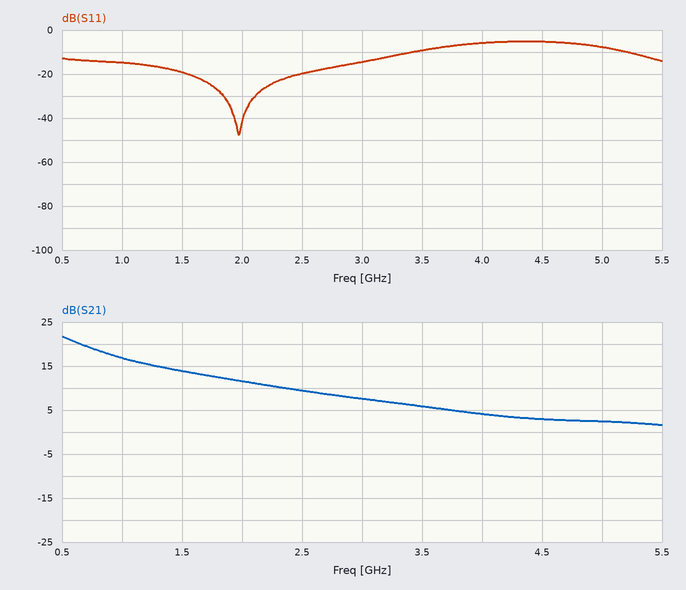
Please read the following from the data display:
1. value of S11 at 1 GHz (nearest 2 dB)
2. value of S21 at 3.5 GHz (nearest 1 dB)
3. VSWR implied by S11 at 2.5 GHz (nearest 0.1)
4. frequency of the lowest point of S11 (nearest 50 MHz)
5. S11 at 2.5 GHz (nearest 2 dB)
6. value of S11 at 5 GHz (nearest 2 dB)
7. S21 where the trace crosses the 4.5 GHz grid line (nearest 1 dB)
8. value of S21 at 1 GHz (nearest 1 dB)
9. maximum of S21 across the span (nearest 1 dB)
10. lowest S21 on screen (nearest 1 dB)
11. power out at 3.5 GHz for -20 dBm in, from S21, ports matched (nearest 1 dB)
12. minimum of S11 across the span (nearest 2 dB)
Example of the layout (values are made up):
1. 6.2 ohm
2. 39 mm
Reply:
1. -14 dB
2. 6 dB
3. 1.2
4. 1.95 GHz
5. -20 dB
6. -8 dB
7. 3 dB
8. 17 dB
9. 22 dB
10. 2 dB
11. -14 dBm
12. -48 dB
